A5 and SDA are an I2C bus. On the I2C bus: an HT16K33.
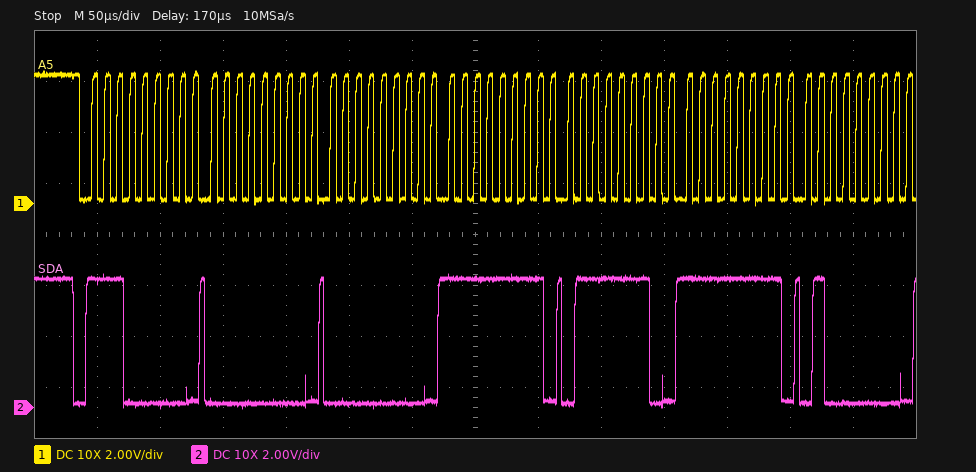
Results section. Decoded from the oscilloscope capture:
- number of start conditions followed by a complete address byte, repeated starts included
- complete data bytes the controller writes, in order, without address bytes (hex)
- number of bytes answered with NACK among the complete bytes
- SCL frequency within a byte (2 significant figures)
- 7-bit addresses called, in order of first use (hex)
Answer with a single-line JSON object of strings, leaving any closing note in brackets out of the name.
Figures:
{"number of start conditions followed by a complete address byte, repeated starts included": "1", "complete data bytes the controller writes, in order, without address bytes": "00 00 FF 7E FF 40", "number of bytes answered with NACK among the complete bytes": "0", "SCL frequency within a byte": "100 kHz", "7-bit addresses called, in order of first use": "0x70"}
